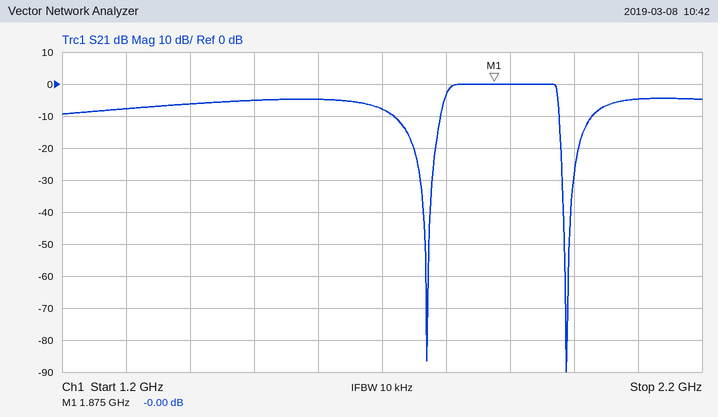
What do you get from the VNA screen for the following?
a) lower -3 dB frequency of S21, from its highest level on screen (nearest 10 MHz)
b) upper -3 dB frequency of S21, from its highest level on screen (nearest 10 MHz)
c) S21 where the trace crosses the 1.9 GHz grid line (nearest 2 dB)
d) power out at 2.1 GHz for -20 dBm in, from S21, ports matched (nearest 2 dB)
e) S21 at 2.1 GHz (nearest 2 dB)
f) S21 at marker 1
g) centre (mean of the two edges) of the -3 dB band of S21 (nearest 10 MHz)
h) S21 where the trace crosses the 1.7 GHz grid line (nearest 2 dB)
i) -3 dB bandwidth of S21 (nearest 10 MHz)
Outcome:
1.80 GHz
1.97 GHz
0 dB
-24 dBm
-4 dB
-0.00 dB
1.89 GHz
-8 dB
170 MHz
